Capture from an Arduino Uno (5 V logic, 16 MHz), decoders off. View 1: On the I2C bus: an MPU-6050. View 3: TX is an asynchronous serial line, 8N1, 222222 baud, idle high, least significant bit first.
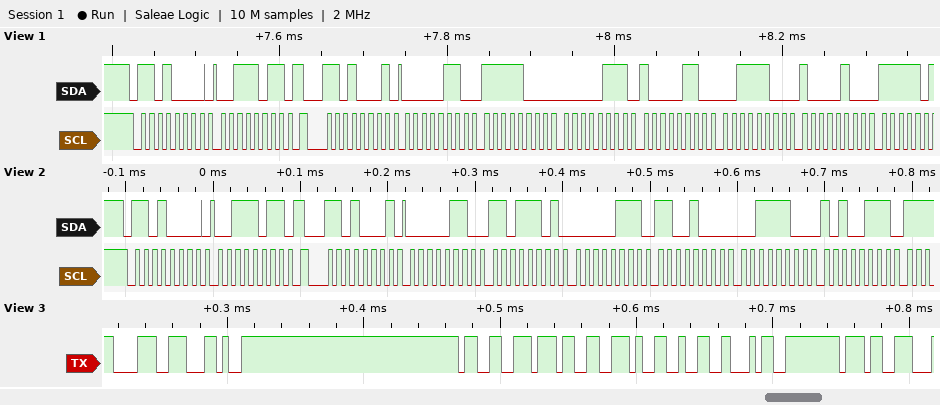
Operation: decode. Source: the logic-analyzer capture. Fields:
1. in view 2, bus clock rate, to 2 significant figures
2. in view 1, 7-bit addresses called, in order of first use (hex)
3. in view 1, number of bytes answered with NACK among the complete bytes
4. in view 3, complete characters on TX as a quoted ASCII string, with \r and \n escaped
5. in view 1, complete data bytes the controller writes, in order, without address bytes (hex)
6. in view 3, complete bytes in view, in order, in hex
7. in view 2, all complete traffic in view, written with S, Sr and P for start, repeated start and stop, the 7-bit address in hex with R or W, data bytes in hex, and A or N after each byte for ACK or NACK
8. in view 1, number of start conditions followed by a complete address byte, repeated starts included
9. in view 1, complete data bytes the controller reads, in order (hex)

100 kHz
0x68
0
"8,37.247"
3B
38 2C 33 37 2E 32 34 37
S 68W A 3B A Sr 68R A 06 A DD A 07 A C8 A 3C A A7 A
2
06 F8 07 86 3C 84
